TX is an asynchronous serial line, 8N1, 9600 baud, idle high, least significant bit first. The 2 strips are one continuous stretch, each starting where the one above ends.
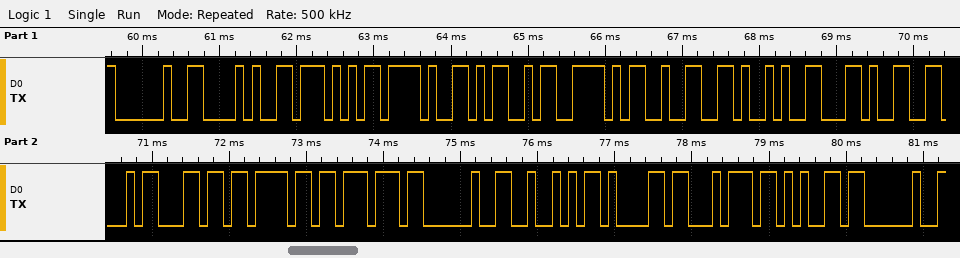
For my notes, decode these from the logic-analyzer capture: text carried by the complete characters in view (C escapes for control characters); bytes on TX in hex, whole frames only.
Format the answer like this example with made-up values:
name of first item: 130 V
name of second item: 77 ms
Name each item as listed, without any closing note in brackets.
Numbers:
text carried by the complete characters in view: " (W/M^2),Flow Rate "
bytes on TX in hex, whole frames only: 20 28 57 2F 4D 5E 32 29 2C 46 6C 6F 77 20 52 61 74 65 20
